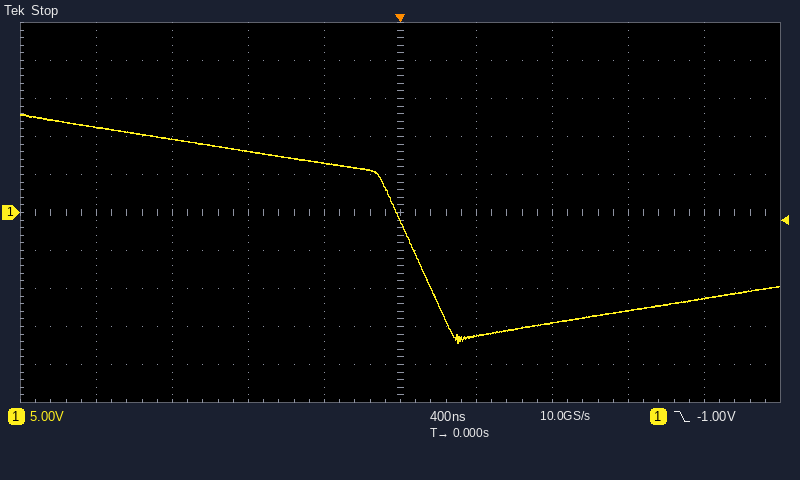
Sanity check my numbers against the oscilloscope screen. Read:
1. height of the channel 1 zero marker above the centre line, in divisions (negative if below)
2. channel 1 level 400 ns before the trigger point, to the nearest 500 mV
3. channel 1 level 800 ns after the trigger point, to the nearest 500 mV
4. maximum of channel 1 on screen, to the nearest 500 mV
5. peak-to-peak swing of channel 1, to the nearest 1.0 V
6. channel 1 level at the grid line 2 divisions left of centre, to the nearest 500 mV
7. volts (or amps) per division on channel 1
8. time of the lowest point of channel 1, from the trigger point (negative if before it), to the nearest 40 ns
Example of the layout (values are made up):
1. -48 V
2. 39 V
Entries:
1. 0.0 div
2. 6.5 V
3. -14.5 V
4. 13.0 V
5. 30.0 V
6. 8.0 V
7. 5 V
8. +320 ns
